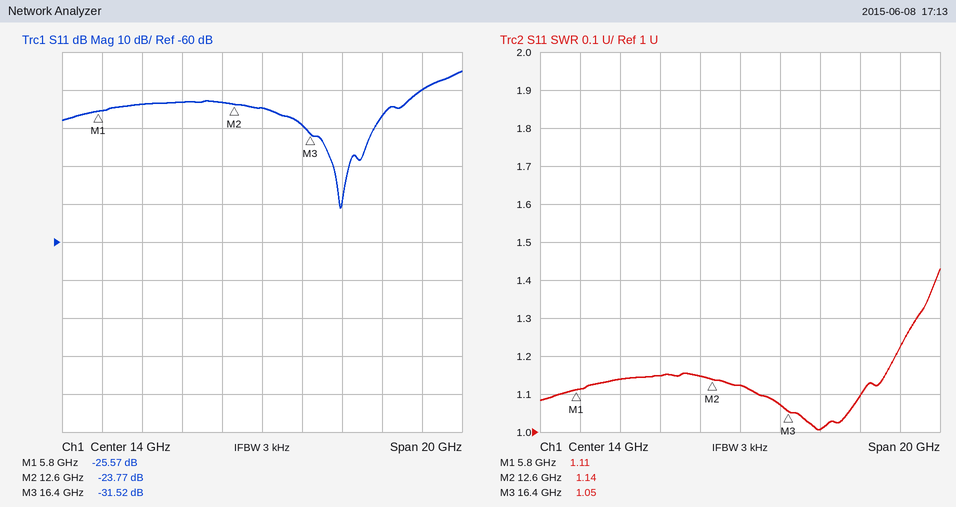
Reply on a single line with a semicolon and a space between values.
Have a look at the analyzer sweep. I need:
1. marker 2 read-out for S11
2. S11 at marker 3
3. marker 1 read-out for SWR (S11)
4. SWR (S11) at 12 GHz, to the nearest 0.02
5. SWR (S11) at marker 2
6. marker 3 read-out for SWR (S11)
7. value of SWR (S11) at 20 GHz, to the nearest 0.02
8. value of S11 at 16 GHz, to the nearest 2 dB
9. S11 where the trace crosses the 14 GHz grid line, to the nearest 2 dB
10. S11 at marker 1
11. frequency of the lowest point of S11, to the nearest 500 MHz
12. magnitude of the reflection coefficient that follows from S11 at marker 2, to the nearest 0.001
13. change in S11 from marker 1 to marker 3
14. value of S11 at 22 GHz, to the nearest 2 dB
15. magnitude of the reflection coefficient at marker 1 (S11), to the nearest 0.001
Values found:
-23.77 dB; -31.52 dB; 1.11; 1.14; 1.14; 1.05; 1.10; -30 dB; -24 dB; -25.57 dB; 18.0 GHz; 0.065; -5.95 dB; -20 dB; 0.053
